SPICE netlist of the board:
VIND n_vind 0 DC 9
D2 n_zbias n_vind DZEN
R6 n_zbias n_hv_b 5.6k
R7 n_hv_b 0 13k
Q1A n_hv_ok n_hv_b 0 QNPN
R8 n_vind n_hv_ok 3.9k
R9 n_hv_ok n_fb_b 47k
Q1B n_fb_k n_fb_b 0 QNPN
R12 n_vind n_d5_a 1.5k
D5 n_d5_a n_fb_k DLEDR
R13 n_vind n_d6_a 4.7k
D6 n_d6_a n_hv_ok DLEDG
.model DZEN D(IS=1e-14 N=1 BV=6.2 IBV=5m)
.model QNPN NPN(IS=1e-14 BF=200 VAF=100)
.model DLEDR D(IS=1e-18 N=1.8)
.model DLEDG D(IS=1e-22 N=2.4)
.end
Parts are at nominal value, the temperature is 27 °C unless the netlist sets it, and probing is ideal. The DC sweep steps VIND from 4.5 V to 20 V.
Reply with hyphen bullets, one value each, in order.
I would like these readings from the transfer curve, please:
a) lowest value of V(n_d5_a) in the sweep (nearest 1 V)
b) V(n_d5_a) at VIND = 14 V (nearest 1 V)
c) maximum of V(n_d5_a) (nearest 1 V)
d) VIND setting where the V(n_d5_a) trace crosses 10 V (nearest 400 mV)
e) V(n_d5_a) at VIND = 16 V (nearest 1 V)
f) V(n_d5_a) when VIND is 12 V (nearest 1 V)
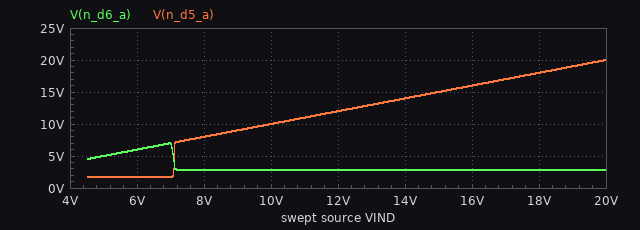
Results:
- 2 V
- 14 V
- 20 V
- 10.0 V
- 16 V
- 12 V
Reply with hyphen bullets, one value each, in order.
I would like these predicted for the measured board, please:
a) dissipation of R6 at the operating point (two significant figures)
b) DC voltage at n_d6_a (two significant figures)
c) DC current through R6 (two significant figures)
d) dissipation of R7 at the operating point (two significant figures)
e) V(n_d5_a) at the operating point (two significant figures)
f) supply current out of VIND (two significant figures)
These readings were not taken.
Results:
- 840 µW
- 2.8 V
- 390 µA
- 37 µW
- 9.0 V
- 4.0 mA
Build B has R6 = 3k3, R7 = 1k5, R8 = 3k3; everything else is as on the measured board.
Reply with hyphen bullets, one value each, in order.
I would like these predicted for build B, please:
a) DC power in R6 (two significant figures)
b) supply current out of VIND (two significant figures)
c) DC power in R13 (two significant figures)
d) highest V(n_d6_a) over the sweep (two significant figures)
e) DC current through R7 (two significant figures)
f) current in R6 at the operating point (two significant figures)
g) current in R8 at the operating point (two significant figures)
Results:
- 1.4 mW
- 4.7 mA
- 8.1 mW
- 8.2 V
- 460 µA
- 650 µA
- 2.7 mA
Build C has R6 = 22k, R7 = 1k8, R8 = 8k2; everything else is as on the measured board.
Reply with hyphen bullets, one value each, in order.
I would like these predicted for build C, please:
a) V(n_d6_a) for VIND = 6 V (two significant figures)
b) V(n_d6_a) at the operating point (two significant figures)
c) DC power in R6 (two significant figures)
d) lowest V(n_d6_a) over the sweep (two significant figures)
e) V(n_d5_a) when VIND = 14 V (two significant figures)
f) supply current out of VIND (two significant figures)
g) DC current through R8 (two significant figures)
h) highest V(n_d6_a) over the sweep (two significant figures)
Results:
- 6.0 V
- 9.0 V
- 330 µW
- 2.9 V
- 1.8 V
- 5.1 mA
- 150 µA
- 14 V
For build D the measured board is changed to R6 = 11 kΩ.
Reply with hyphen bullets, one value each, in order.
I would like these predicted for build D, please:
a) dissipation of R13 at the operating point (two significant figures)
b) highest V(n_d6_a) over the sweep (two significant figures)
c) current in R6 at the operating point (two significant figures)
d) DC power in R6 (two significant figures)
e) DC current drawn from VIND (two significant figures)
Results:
- 8.1 mW
- 7.3 V
- 200 µA
- 440 µW
- 3.8 mA
